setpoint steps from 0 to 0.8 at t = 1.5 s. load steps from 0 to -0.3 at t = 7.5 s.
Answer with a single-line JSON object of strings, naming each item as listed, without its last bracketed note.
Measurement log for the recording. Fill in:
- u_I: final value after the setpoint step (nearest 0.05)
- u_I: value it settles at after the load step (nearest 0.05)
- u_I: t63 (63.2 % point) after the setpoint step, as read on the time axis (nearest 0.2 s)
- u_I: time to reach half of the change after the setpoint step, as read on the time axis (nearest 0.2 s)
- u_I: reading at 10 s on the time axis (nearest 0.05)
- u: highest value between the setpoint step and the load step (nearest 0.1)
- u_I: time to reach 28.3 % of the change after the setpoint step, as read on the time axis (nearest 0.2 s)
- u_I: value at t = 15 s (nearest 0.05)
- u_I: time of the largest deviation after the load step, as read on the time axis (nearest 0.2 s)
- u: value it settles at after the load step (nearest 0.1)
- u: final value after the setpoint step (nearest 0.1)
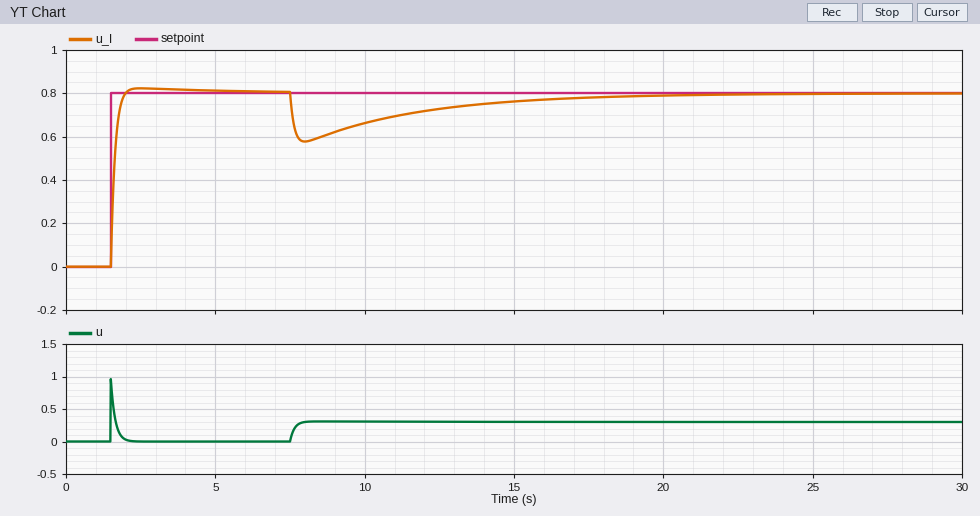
{"u_I: final value after the setpoint step": "0.80", "u_I: value it settles at after the load step": "0.80", "u_I: t63 (63.2 % point) after the setpoint step, as read on the time axis": "1.6 s", "u_I: time to reach half of the change after the setpoint step, as read on the time axis": "1.6 s", "u_I: reading at 10 s on the time axis": "0.65", "u: highest value between the setpoint step and the load step": "1.0", "u_I: time to reach 28.3 % of the change after the setpoint step, as read on the time axis": "1.6 s", "u_I: value at t = 15 s": "0.75", "u_I: time of the largest deviation after the load step, as read on the time axis": "8.0 s", "u: value it settles at after the load step": "0.3", "u: final value after the setpoint step": "0.0"}
